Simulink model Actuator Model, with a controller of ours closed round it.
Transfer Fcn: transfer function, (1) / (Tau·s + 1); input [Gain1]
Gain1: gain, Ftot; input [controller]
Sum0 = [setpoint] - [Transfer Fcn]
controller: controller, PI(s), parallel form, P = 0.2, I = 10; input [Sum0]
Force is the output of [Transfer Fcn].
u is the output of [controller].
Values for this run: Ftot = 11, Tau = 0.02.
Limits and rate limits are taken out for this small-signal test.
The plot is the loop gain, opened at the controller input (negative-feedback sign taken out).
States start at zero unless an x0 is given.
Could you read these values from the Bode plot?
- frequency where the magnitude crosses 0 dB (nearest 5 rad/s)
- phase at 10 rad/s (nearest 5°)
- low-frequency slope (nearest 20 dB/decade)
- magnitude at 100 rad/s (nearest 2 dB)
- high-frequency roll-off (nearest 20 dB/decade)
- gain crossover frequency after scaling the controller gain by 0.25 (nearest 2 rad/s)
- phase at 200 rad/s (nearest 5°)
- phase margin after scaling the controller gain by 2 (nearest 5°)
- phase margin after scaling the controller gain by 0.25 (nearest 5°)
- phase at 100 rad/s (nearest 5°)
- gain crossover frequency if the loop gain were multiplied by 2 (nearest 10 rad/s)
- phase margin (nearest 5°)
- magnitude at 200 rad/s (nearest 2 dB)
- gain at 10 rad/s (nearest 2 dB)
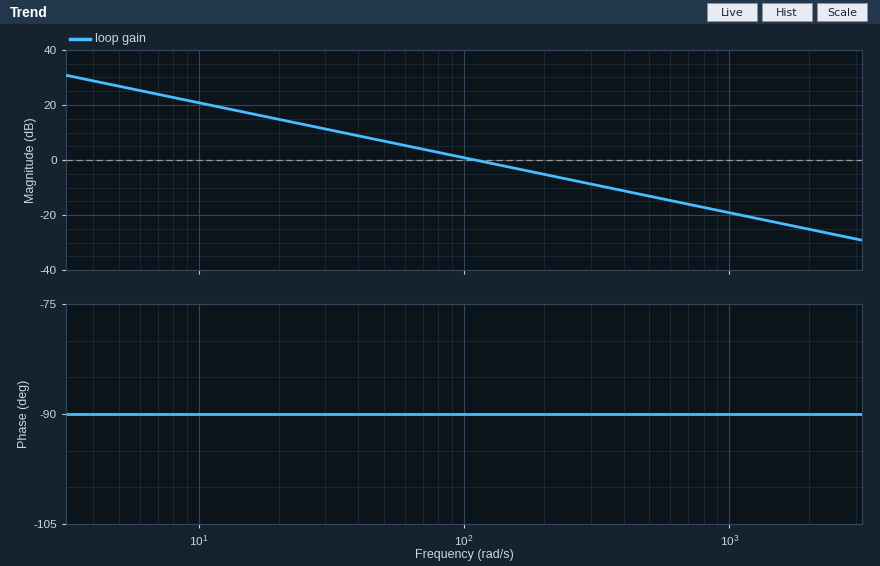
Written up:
110 rad/s
-90°
-20 dB/decade
0 dB
-20 dB/decade
28 rad/s
-90°
90°
90°
-90°
220 rad/s
90°
-6 dB
20 dB
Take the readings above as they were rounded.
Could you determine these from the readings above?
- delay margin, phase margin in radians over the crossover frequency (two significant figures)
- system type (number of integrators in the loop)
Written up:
0.014 s
1
